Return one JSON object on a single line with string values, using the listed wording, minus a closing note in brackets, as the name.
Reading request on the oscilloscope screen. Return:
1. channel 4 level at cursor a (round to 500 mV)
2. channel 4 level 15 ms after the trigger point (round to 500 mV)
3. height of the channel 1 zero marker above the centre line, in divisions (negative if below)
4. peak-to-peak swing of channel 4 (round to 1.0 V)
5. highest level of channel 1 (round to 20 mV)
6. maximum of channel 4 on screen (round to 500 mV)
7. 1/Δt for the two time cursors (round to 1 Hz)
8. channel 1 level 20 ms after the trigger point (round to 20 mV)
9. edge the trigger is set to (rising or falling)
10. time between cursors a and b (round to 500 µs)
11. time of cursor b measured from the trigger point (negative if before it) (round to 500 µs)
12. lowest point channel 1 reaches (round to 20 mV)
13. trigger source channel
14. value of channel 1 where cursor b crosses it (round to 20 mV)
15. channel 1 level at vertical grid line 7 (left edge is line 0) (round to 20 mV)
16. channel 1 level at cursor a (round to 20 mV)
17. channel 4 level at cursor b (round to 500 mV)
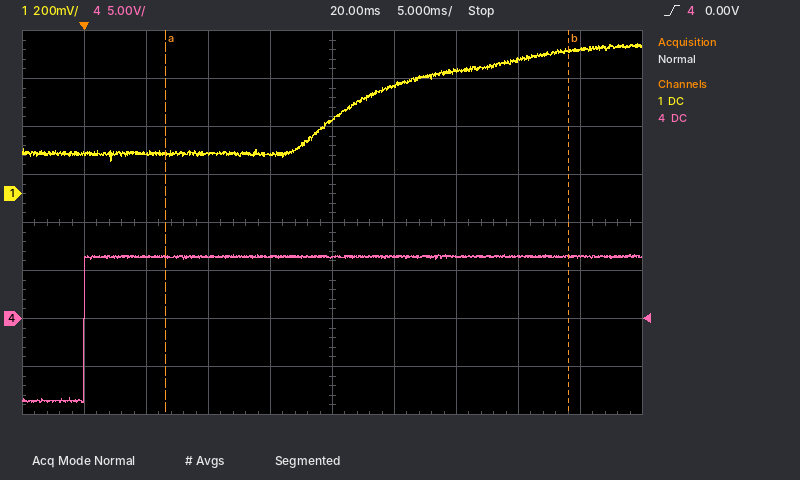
{"channel 4 level at cursor a": "6.5 V", "channel 4 level 15 ms after the trigger point": "6.5 V", "height of the channel 1 zero marker above the centre line, in divisions": "+0.6 div", "peak-to-peak swing of channel 4": "15.0 V", "highest level of channel 1": "620 mV", "maximum of channel 4 on screen": "6.5 V", "1/Δt for the two time cursors": "31 Hz", "channel 1 level 20 ms after the trigger point": "300 mV", "edge the trigger is set to": "rising", "time between cursors a and b": "32.5 ms", "time of cursor b measured from the trigger point (negative if before it)": "+39.0 ms", "lowest point channel 1 reaches": "140 mV", "trigger source channel": "channel 4", "value of channel 1 where cursor b crosses it": "600 mV", "channel 1 level at vertical grid line 7 (left edge is line 0)": "520 mV", "channel 1 level at cursor a": "160 mV", "channel 4 level at cursor b": "6.5 V"}
